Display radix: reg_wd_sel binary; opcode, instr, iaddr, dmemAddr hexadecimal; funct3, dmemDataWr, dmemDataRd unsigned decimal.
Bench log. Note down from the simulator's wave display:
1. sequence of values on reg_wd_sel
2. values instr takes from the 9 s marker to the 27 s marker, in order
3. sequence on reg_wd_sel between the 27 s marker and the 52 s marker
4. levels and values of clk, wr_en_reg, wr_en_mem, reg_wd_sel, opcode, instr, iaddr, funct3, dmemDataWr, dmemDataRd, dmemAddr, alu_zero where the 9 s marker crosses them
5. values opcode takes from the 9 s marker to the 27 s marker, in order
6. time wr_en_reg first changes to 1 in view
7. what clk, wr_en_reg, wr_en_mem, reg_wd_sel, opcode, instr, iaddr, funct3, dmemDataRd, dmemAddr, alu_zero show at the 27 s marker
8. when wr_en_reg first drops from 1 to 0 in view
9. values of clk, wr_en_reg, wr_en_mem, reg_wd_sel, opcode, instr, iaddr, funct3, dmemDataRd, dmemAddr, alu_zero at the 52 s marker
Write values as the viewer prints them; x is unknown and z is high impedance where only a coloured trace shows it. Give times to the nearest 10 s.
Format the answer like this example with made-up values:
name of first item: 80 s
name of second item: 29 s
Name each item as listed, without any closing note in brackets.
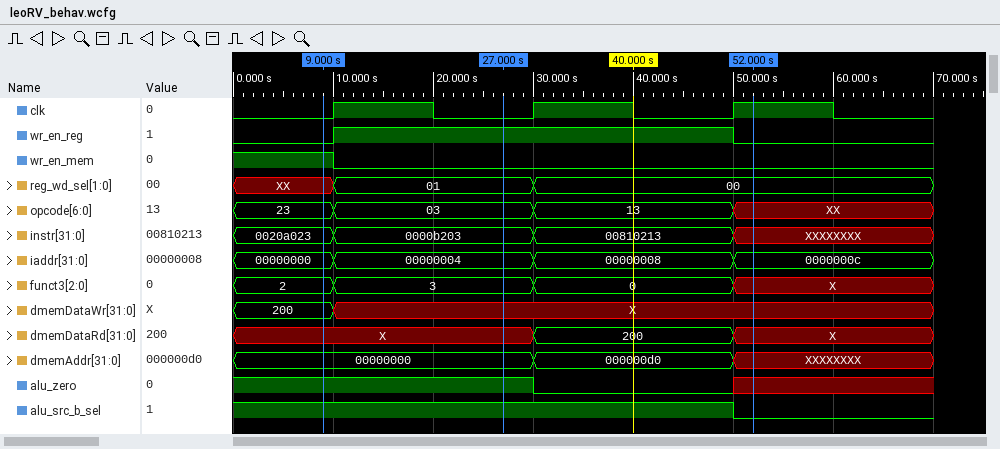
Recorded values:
sequence of values on reg_wd_sel: XX, 01, 00
values instr takes from the 9 s marker to the 27 s marker, in order: 0020a023, 0000b203
sequence on reg_wd_sel between the 27 s marker and the 52 s marker: 01, 00
levels and values of clk, wr_en_reg, wr_en_mem, reg_wd_sel, opcode, instr, iaddr, funct3, dmemDataWr, dmemDataRd, dmemAddr, alu_zero where the 9 s marker crosses them: clk=0, wr_en_reg=0, wr_en_mem=1, reg_wd_sel=XX, opcode=23, instr=0020a023, iaddr=00000000, funct3=2, dmemDataWr=200, dmemDataRd=X, dmemAddr=00000000, alu_zero=1
values opcode takes from the 9 s marker to the 27 s marker, in order: 23, 03
time wr_en_reg first changes to 1 in view: 10 s
what clk, wr_en_reg, wr_en_mem, reg_wd_sel, opcode, instr, iaddr, funct3, dmemDataRd, dmemAddr, alu_zero show at the 27 s marker: clk=0, wr_en_reg=1, wr_en_mem=0, reg_wd_sel=01, opcode=03, instr=0000b203, iaddr=00000004, funct3=3, dmemDataRd=X, dmemAddr=00000000, alu_zero=1
when wr_en_reg first drops from 1 to 0 in view: 50 s
values of clk, wr_en_reg, wr_en_mem, reg_wd_sel, opcode, instr, iaddr, funct3, dmemDataRd, dmemAddr, alu_zero at the 52 s marker: clk=1, wr_en_reg=0, wr_en_mem=0, reg_wd_sel=00, opcode=XX, instr=XXXXXXXX, iaddr=0000000c, funct3=X, dmemDataRd=X, dmemAddr=XXXXXXXX, alu_zero=x
